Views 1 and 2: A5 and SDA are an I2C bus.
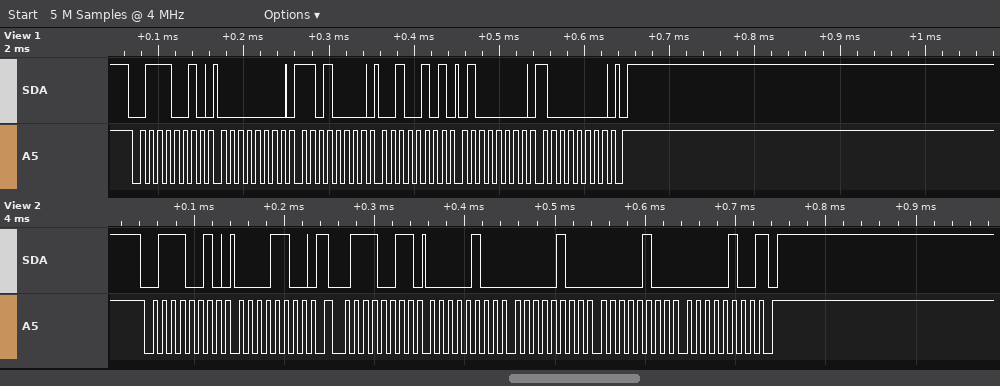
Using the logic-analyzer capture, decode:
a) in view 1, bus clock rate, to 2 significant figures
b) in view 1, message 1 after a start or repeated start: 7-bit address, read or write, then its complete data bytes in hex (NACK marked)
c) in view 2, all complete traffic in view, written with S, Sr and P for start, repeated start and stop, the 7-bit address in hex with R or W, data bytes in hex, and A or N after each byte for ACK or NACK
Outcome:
100 kHz
0x39 write: 00 D0 25 40 80
S 39W A 0C A Sr 39R A 04 A 04 A 04 A 04 N P
